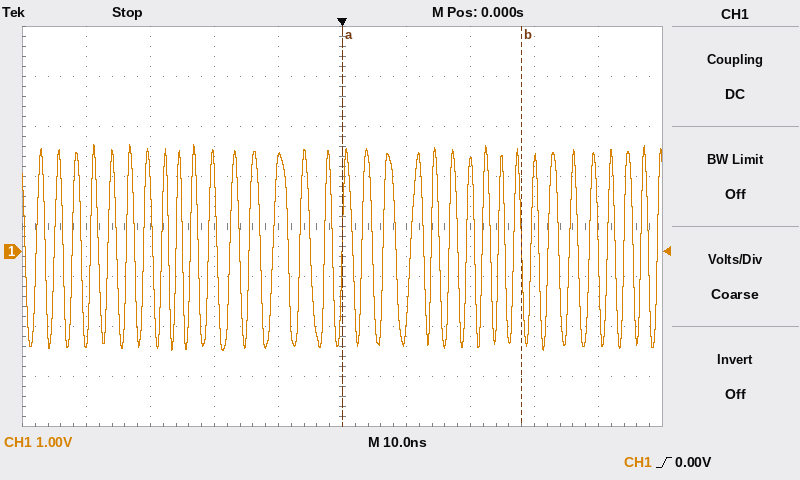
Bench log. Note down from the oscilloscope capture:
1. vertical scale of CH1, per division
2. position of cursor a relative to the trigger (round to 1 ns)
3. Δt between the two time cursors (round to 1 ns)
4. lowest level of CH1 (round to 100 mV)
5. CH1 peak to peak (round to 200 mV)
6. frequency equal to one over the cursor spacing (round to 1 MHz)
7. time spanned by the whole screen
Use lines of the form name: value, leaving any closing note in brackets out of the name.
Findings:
vertical scale of CH1, per division: 1 V
position of cursor a relative to the trigger: 0 ns
Δt between the two time cursors: 28 ns
lowest level of CH1: -2.0 V
CH1 peak to peak: 4.2 V
frequency equal to one over the cursor spacing: 36 MHz
time spanned by the whole screen: 100 ns
